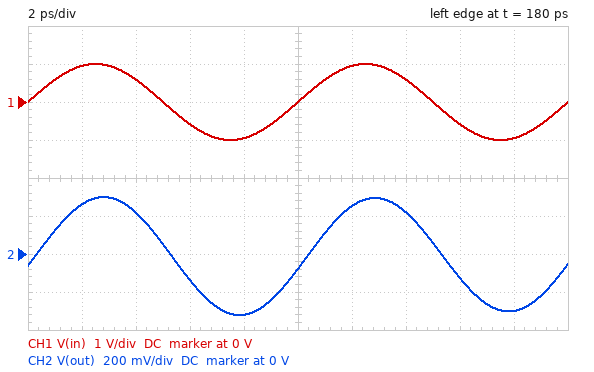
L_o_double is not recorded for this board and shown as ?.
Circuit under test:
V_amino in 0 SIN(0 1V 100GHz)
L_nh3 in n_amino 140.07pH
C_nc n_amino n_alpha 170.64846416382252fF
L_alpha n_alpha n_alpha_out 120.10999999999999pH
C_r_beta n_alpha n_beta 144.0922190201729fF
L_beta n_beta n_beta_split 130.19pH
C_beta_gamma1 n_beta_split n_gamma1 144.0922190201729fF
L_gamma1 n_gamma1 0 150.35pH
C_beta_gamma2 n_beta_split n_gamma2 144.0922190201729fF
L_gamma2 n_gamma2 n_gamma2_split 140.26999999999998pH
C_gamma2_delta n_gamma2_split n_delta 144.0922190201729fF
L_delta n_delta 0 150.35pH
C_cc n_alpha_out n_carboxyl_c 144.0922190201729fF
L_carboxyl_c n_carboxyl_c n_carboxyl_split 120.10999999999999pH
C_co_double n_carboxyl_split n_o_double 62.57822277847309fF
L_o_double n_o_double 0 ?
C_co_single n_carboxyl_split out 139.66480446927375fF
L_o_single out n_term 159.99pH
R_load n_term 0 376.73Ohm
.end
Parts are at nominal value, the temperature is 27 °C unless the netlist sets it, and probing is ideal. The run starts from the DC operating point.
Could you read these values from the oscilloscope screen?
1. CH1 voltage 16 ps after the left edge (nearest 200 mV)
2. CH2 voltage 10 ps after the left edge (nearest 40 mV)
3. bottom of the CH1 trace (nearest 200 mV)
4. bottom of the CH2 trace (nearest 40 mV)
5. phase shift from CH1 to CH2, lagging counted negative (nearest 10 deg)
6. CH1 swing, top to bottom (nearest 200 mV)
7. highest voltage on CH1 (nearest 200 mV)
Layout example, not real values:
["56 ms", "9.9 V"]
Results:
["-600 mV", "-80 mV", "-1.0 V", "-320 mV", "-10 deg", "2.0 V", "1.0 V"]
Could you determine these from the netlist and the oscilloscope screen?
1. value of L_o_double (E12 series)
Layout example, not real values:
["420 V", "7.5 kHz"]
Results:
["390 pH"]
